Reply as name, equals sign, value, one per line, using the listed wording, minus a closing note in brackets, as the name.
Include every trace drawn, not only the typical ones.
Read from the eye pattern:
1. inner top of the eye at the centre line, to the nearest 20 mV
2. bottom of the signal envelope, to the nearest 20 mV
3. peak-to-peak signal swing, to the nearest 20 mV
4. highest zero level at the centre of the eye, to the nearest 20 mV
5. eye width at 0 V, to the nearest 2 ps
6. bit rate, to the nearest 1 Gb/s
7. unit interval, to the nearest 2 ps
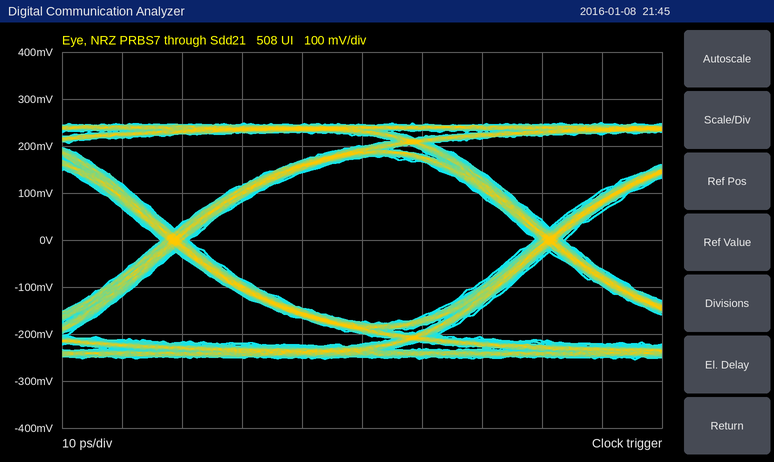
inner top of the eye at the centre line, to the nearest 20 mV = 180 mV
bottom of the signal envelope, to the nearest 20 mV = -260 mV
peak-to-peak signal swing, to the nearest 20 mV = 500 mV
highest zero level at the centre of the eye, to the nearest 20 mV = -180 mV
eye width at 0 V, to the nearest 2 ps = 58 ps
bit rate, to the nearest 1 Gb/s = 16 Gb/s
unit interval, to the nearest 2 ps = 62 ps
